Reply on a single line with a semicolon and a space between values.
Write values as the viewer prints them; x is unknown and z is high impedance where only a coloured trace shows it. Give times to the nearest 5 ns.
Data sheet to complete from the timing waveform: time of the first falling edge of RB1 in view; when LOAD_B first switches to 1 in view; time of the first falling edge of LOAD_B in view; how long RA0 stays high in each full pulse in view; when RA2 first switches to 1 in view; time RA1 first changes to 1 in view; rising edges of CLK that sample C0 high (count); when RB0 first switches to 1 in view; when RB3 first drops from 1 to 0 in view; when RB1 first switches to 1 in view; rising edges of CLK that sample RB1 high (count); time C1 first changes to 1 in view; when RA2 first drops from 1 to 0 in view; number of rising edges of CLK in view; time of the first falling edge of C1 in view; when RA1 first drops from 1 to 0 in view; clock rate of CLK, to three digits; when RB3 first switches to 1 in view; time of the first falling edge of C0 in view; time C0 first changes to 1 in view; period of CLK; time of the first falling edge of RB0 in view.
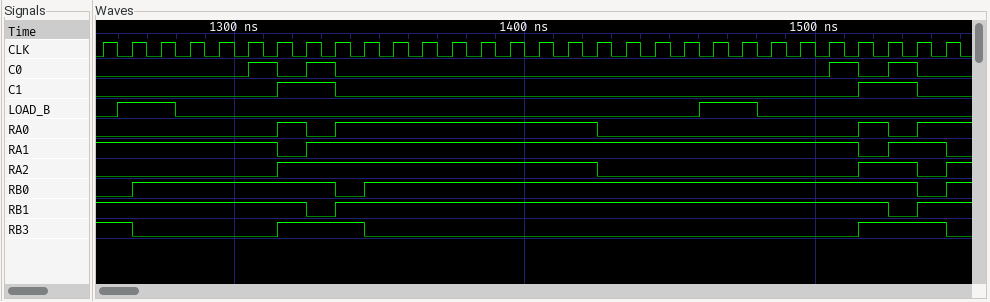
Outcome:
1325 ns; 1260 ns; 1280 ns; 10 ns, 90 ns, 10 ns; 1315 ns; 1325 ns; 4; 1265 ns; 1265 ns; 1335 ns; 28; 1315 ns; 1425 ns; 30; 1335 ns; 1315 ns; 100 MHz; 1315 ns; 1315 ns; 1305 ns; 10 ns; 1335 ns
